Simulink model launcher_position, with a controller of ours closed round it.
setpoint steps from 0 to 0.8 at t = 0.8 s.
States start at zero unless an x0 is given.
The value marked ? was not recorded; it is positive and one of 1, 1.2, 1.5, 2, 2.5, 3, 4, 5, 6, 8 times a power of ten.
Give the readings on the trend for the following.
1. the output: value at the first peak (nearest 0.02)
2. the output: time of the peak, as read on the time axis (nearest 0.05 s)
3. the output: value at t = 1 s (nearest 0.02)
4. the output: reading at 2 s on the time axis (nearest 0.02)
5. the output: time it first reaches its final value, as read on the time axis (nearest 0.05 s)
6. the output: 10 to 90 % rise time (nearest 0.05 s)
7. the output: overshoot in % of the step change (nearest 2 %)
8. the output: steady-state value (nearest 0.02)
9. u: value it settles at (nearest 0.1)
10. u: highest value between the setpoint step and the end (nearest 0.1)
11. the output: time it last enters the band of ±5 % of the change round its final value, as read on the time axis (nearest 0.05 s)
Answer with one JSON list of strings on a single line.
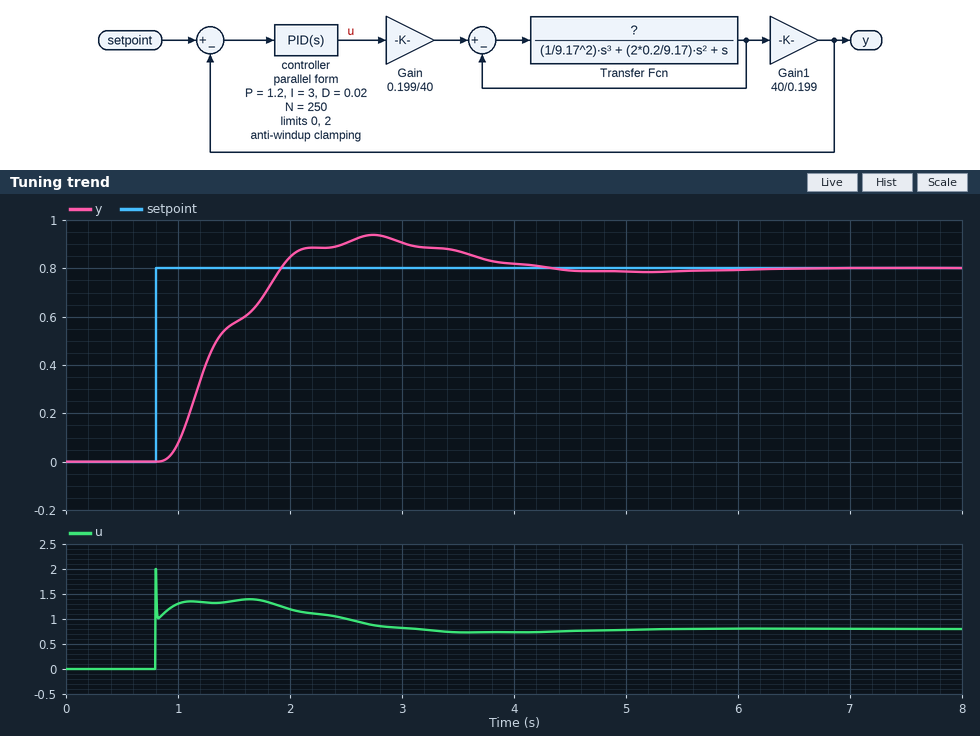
["0.94", "2.75 s", "0.08", "0.84", "1.90 s", "0.80 s", "18 %", "0.80", "0.8", "2.0", "3.70 s"]
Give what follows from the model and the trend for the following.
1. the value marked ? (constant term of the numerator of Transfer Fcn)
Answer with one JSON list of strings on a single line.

["0.8"]
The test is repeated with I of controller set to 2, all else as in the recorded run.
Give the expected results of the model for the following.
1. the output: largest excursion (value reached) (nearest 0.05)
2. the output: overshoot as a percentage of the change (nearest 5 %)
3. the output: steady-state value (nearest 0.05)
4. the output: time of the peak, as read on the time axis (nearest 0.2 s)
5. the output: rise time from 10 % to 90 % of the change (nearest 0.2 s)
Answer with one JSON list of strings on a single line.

["0.85", "10 %", "0.80", "3.4 s", "1.0 s"]
